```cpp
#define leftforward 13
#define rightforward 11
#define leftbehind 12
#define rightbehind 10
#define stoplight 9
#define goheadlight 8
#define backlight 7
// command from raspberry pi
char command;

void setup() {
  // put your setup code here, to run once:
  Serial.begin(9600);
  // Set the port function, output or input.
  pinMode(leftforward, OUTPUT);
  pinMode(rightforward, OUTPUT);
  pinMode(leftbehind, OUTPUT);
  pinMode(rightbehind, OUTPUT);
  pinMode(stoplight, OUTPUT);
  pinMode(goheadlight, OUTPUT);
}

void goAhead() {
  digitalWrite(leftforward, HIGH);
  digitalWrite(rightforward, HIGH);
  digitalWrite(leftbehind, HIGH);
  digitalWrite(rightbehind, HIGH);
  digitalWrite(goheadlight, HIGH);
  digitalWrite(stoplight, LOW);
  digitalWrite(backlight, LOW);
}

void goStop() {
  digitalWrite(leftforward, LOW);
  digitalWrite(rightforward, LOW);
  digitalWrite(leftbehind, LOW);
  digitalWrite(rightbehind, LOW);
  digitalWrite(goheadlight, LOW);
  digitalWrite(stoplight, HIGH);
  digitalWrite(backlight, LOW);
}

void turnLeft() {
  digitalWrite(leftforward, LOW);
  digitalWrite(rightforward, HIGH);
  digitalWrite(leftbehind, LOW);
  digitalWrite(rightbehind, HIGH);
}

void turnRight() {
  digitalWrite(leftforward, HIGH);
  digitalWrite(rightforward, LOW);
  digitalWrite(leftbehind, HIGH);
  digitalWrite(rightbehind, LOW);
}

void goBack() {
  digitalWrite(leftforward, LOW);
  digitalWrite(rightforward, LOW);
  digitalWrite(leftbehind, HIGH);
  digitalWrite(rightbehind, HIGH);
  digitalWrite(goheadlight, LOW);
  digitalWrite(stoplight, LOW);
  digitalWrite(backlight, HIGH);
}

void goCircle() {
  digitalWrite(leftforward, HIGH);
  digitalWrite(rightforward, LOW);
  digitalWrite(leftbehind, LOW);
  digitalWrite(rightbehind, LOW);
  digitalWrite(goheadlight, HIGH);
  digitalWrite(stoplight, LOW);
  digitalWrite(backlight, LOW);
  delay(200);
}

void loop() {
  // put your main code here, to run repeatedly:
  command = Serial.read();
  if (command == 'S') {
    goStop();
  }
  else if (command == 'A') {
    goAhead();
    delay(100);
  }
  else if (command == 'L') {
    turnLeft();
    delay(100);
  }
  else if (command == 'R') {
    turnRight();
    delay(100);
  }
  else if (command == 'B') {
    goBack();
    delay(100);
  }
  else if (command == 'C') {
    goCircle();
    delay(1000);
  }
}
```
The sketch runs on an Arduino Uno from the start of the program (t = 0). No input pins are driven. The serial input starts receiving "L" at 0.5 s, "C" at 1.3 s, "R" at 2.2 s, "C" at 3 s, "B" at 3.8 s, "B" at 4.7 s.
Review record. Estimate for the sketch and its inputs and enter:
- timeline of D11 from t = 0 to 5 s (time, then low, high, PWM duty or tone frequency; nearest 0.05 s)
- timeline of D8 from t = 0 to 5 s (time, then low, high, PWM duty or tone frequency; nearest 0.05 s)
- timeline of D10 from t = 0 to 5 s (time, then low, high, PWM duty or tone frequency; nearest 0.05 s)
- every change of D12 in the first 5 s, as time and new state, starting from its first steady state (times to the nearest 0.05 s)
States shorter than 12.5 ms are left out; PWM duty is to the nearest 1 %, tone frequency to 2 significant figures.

0 s low; 0.5 s high; 1.3 s low
0 s low; 1.3 s high; 4.2 s low
0 s low; 0.5 s high; 1.3 s low; 4.2 s high
0 s low; 2.5 s high; 3 s low; 4.2 s high
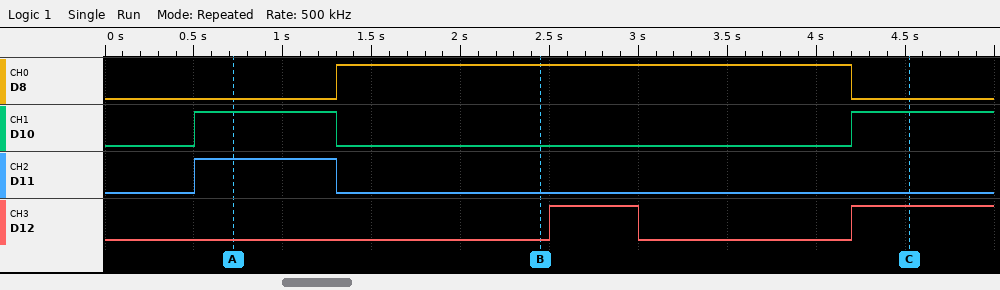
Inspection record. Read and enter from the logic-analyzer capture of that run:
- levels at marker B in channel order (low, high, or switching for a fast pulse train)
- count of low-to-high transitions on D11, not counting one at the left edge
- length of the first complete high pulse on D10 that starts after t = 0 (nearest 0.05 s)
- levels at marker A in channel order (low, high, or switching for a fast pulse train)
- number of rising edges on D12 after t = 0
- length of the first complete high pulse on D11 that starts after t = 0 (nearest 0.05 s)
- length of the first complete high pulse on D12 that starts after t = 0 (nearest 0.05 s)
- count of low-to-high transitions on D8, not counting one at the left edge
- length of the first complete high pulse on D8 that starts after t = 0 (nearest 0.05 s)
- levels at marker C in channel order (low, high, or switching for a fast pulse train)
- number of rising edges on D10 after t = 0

D8 high, D10 low, D11 low, D12 low
1
0.80 s
D8 low, D10 high, D11 high, D12 low
2
0.80 s
0.50 s
1
2.90 s
D8 low, D10 high, D11 low, D12 high
2
